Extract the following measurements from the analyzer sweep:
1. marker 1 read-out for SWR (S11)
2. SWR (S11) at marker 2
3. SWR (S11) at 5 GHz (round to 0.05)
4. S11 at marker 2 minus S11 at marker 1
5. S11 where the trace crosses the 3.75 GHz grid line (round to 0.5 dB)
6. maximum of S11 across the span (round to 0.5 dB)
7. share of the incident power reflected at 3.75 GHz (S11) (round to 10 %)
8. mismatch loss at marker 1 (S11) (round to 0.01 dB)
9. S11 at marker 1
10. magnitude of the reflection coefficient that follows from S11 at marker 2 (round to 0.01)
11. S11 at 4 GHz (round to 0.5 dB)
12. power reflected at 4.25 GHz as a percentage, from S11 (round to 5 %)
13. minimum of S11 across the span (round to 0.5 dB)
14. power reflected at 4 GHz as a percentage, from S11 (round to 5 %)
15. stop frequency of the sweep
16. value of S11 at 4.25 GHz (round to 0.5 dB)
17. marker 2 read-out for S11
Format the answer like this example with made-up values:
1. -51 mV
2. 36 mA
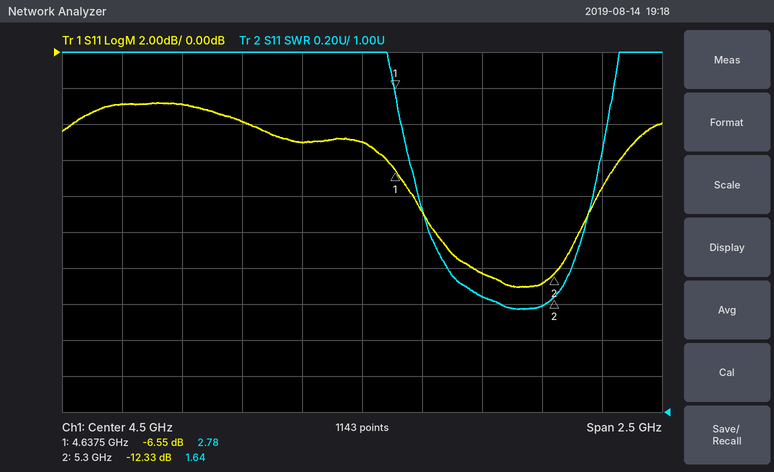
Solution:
1. 2.78
2. 1.64
3. 1.65
4. -5.78 dB
5. -3.0 dB
6. -3.0 dB
7. 50 %
8. 1.09 dB
9. -6.55 dB
10. 0.24
11. -4.0 dB
12. 30 %
13. -13.0 dB
14. 40 %
15. 5.75 GHz
16. -5.0 dB
17. -12.33 dB
